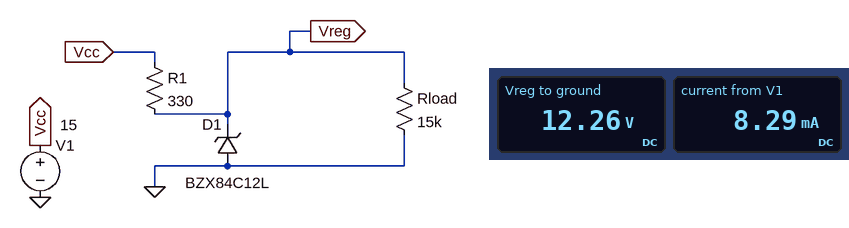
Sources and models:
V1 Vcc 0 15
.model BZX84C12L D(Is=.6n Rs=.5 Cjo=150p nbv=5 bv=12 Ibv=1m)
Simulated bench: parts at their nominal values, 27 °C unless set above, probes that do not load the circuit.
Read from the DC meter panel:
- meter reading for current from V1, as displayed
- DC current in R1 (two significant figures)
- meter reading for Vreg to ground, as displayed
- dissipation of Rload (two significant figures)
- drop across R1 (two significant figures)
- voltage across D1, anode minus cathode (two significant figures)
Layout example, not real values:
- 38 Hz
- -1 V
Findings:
- 8.29 mA
- 8.3 mA
- 12.26 V
- 10 mW
- 2.7 V
- -12 V
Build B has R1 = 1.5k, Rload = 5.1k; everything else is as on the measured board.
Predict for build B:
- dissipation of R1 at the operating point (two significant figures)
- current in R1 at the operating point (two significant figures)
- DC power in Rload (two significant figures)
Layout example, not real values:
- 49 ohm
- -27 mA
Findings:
- 7.9 mW
- 2.3 mA
- 26 mW
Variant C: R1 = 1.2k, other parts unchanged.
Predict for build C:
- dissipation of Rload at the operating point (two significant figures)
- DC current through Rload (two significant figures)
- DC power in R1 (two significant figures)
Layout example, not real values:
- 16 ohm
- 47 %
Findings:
- 9.7 mW
- 800 µA
- 7.2 mW
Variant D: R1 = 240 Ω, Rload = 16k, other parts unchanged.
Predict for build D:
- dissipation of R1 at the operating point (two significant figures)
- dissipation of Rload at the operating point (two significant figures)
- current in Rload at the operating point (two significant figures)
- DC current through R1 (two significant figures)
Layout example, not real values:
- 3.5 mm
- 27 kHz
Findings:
- 30 mW
- 9.5 mW
- 770 µA
- 11 mA
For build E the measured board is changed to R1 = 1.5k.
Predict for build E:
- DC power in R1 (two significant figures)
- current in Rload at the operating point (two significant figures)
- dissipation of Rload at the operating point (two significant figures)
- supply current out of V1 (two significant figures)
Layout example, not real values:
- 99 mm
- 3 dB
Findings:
- 5.9 mW
- 800 µA
- 9.6 mW
- 2.0 mA
